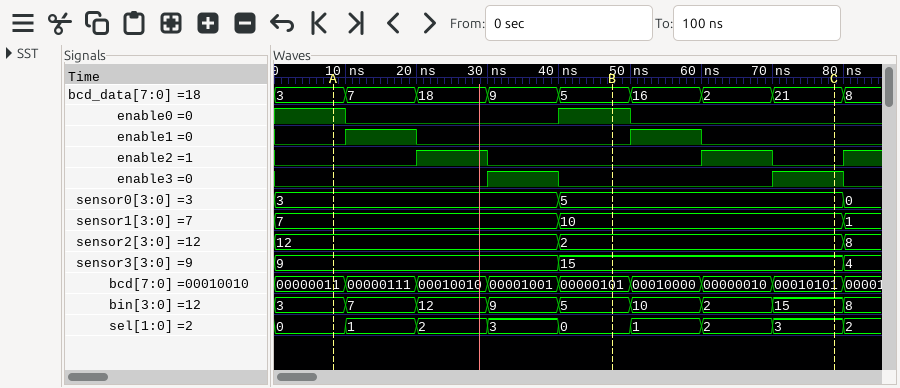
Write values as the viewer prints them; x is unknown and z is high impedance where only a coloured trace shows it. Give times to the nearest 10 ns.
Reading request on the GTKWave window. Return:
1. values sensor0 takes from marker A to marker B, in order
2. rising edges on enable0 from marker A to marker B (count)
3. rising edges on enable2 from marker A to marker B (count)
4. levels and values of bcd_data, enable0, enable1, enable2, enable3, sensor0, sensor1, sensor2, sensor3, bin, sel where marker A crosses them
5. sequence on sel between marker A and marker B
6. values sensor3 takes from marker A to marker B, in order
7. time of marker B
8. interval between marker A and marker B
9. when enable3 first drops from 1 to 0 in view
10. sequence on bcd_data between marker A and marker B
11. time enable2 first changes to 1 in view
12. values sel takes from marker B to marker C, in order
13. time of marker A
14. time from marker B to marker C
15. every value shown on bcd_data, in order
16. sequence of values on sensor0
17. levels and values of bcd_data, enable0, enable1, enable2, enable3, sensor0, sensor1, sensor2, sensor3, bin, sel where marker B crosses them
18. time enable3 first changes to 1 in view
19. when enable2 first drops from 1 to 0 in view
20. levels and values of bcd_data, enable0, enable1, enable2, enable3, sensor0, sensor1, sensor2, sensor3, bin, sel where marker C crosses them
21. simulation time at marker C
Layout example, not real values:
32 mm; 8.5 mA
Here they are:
3, 5; 1; 1; bcd_data=3, enable0=1, enable1=0, enable2=0, enable3=0, sensor0=3, sensor1=7, sensor2=12, sensor3=9, bin=3, sel=0; 0, 1, 2, 3, 0; 9, 15; 50 ns; 40 ns; 40 ns; 3, 7, 18, 9, 5; 20 ns; 0, 1, 2, 3; 10 ns; 30 ns; 3, 7, 18, 9, 5, 16, 2, 21, 8; 3, 5, 0; bcd_data=5, enable0=1, enable1=0, enable2=0, enable3=0, sensor0=5, sensor1=10, sensor2=2, sensor3=15, bin=5, sel=0; 30 ns; 30 ns; bcd_data=21, enable0=0, enable1=0, enable2=0, enable3=1, sensor0=5, sensor1=10, sensor2=2, sensor3=15, bin=15, sel=3; 80 ns
